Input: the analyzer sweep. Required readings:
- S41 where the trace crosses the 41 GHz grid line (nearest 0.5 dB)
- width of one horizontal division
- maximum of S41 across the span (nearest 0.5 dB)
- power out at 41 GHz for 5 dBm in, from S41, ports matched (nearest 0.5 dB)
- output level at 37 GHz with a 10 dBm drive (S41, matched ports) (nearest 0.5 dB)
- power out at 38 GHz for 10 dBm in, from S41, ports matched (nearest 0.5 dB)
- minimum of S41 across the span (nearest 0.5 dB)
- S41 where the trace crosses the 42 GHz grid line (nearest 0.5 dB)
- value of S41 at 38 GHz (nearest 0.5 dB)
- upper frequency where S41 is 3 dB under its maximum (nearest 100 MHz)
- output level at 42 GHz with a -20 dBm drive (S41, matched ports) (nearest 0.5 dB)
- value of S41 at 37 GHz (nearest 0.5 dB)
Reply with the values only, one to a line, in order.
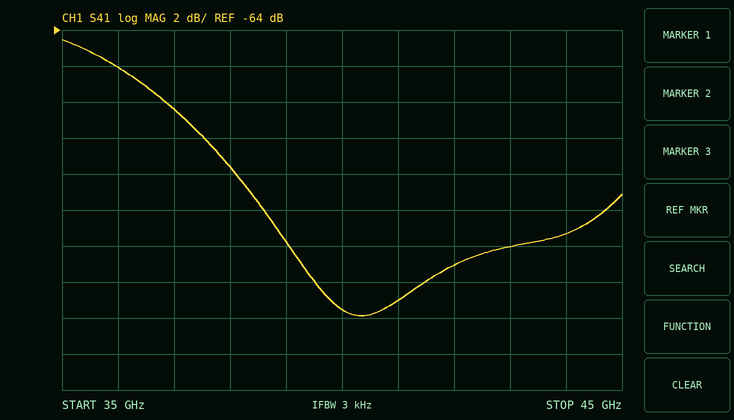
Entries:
-79.0 dB
1 GHz
-64.5 dB
-74.0 dBm
-58.5 dBm
-61.5 dBm
-80.0 dB
-77.0 dB
-71.5 dB
36.7 GHz
-97.0 dBm
-68.5 dB
